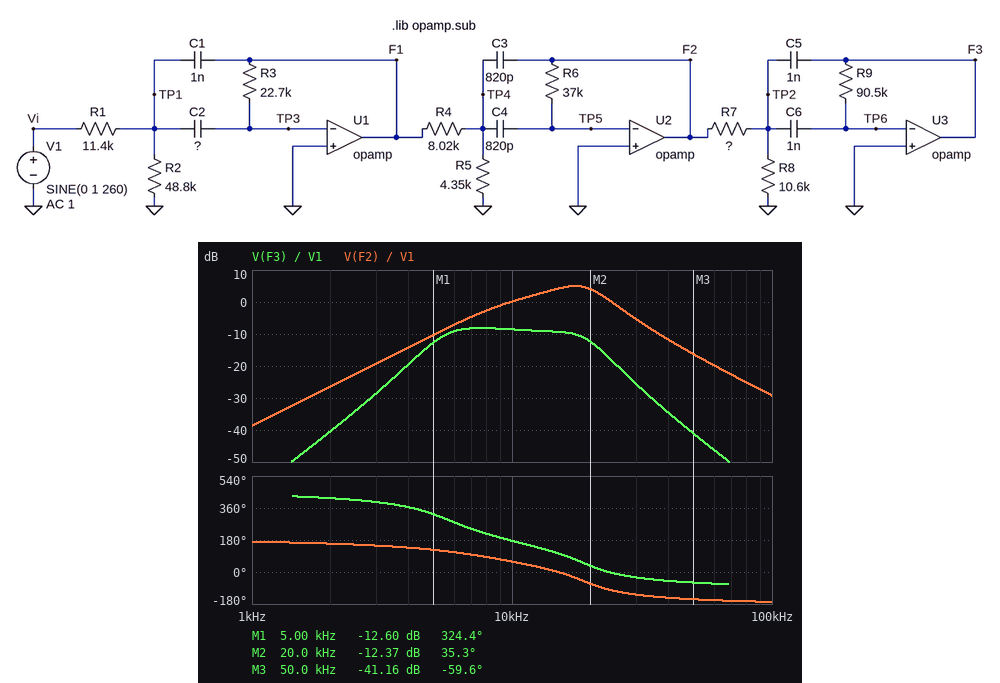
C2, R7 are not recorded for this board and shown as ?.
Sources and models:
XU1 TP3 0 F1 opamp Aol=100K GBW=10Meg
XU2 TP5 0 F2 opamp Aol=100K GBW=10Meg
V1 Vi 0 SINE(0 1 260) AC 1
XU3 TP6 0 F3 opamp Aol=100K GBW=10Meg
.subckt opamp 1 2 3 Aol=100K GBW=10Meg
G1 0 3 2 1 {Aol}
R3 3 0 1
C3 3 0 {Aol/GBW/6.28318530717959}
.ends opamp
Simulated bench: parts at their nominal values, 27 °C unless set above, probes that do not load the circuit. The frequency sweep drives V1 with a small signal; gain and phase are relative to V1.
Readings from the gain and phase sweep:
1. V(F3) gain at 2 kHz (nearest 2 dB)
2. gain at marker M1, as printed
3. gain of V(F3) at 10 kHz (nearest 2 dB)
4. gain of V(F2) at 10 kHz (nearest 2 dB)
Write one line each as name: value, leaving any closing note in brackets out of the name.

V(F3) gain at 2 kHz: -40 dB
gain at marker M1, as printed: -12.60 dB
gain of V(F3) at 10 kHz: -8 dB
gain of V(F2) at 10 kHz: 0 dB
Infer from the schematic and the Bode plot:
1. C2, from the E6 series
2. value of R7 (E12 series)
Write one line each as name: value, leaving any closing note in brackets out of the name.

C2, from the E6 series: 1.5 nF
value of R7: 56 kΩ
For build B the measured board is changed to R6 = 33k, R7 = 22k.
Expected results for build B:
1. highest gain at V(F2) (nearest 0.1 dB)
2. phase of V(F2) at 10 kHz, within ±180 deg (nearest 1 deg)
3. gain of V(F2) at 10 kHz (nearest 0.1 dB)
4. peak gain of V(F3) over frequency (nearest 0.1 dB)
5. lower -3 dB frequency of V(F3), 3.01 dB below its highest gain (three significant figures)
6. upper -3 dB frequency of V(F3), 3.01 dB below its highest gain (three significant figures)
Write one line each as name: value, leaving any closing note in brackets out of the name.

highest gain at V(F2): 3.6 dB
phase of V(F2) at 10 kHz, within ±180 deg: 59 deg
gain of V(F2) at 10 kHz: -1.2 dB
peak gain of V(F3) over frequency: 0 dB
lower -3 dB frequency of V(F3), 3.01 dB below its highest gain: 5.75 kHz
upper -3 dB frequency of V(F3), 3.01 dB below its highest gain: 16.8 kHz
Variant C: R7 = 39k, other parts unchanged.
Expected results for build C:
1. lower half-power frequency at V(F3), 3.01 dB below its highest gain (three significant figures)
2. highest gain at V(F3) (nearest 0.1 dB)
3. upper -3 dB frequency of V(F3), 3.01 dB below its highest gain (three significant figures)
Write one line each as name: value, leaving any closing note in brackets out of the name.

lower half-power frequency at V(F3), 3.01 dB below its highest gain: 5.43 kHz
highest gain at V(F3): -4.7 dB
upper -3 dB frequency of V(F3), 3.01 dB below its highest gain: 18.6 kHz
